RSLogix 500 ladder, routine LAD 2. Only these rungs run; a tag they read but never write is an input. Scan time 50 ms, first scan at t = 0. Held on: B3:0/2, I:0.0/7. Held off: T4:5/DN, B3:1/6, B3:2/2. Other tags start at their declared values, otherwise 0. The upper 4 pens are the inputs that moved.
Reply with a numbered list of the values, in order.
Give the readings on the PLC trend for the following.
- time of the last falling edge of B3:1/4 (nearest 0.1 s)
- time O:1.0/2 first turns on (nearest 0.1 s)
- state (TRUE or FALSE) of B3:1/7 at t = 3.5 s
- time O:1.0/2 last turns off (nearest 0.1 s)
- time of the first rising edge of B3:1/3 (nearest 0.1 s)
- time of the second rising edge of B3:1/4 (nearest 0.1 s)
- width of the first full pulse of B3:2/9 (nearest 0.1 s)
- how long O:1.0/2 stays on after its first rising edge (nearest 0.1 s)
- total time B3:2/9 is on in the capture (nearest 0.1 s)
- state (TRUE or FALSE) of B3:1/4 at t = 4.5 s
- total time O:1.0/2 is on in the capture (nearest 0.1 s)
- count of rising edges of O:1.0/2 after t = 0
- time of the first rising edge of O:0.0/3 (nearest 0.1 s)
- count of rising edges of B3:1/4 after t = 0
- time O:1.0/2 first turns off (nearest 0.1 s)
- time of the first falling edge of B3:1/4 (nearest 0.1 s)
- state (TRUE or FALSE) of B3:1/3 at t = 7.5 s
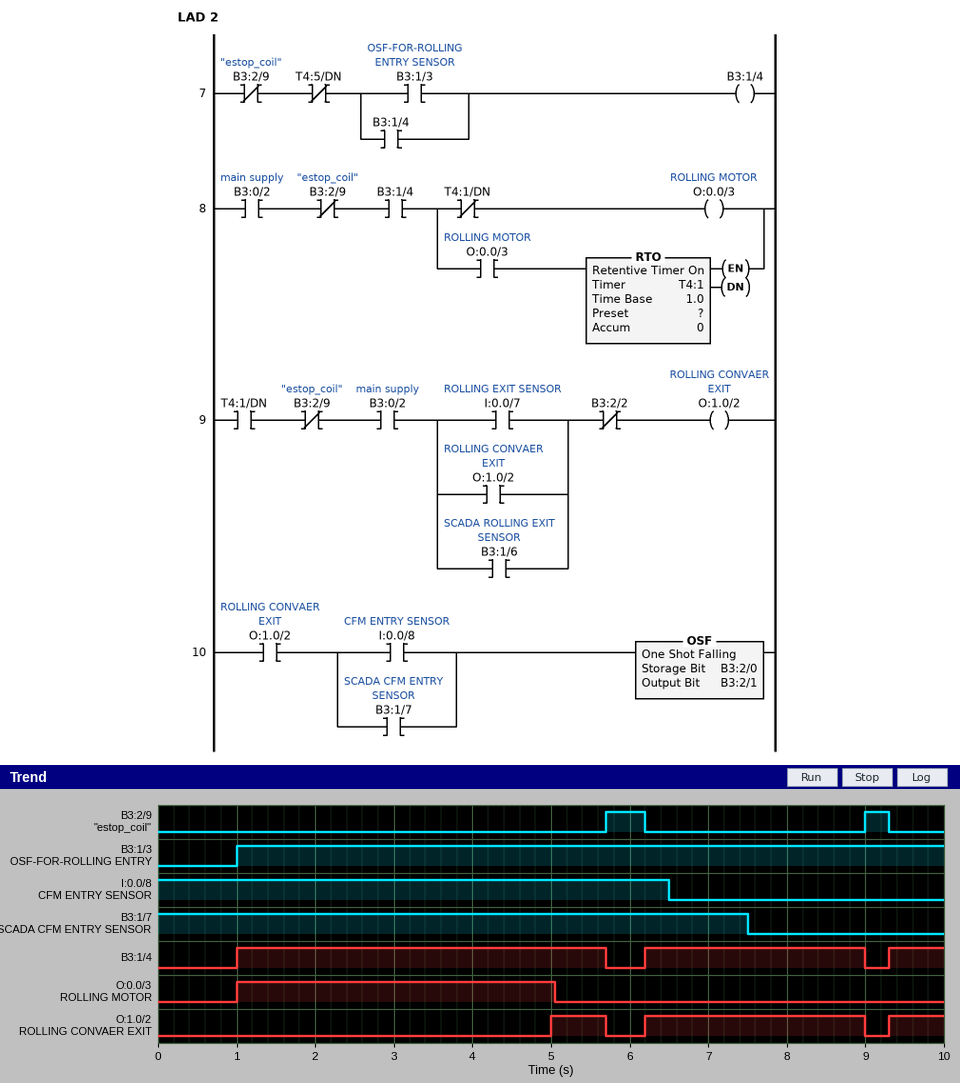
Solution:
1. 9.0 s
2. 5.0 s
3. TRUE
4. 9.0 s
5. 1.0 s
6. 6.2 s
7. 0.5 s
8. 0.7 s
9. 0.8 s
10. TRUE
11. 4.2 s
12. 3
13. 1.0 s
14. 3
15. 5.7 s
16. 5.7 s
17. TRUE
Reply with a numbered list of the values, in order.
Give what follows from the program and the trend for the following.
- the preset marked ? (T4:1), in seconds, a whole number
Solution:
1. 4 s
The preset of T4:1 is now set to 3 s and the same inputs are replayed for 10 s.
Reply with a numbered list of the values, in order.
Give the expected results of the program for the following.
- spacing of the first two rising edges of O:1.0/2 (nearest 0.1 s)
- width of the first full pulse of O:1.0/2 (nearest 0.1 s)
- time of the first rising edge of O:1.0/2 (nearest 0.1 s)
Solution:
1. 2.2 s
2. 1.7 s
3. 4.0 s
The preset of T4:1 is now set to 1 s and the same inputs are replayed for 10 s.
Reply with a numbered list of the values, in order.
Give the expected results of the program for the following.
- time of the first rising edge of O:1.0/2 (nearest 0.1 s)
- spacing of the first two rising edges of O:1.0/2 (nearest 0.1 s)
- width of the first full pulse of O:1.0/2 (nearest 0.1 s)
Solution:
1. 2.0 s
2. 4.2 s
3. 3.7 s
